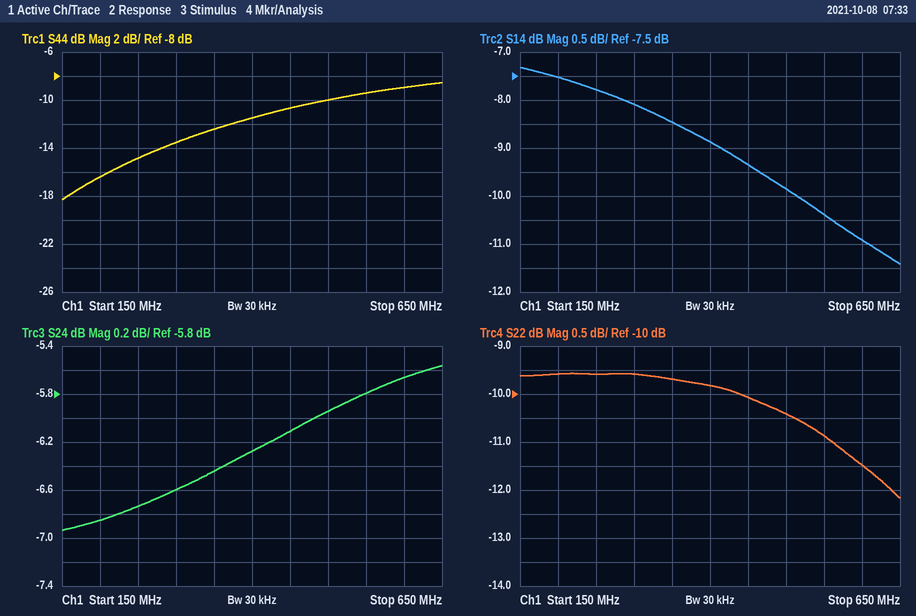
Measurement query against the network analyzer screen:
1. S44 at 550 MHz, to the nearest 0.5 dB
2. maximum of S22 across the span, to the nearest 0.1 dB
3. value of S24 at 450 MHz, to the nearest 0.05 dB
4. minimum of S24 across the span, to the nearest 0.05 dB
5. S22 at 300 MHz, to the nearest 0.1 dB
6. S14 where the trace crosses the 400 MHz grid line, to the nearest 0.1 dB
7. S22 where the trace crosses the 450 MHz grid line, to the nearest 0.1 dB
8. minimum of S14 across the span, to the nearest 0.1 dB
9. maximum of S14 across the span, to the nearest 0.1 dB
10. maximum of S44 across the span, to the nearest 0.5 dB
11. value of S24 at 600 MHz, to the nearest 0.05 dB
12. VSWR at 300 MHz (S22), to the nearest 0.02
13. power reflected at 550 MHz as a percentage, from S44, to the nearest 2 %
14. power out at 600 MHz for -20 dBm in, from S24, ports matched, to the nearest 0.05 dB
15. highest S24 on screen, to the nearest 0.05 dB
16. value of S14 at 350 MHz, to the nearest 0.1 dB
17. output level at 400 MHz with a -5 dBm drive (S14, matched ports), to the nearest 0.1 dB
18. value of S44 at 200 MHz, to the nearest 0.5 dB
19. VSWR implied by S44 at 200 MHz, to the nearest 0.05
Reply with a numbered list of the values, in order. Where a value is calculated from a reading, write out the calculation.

1. -9.5 dB
2. -9.6 dB
3. -6.10 dB
4. -6.95 dB
5. -9.6 dB
6. -8.9 dB
7. -10.1 dB
8. -11.4 dB
9. -7.3 dB
10. -8.5 dB
11. -5.65 dB
12. |Γ| = 10^(-9.6/20) = 0.3311; VSWR = (1 + 0.3311)/(1 − 0.3311) ≈ 1.99, so 2.00 to the nearest 0.02
13. 10^(-9.5/10) ≈ 11.2 %, so 12 % to the nearest 2 %
14. -20 dBm + (-5.65 dB) = -25.65 dBm
15. -5.55 dB
16. -8.5 dB
17. -5 dBm + (-8.9 dB) = -13.9 dBm
18. -16.5 dB
19. |Γ| = 10^(-16.5/20) = 0.1496; VSWR = (1 + 0.1496)/(1 − 0.1496) ≈ 1.35
